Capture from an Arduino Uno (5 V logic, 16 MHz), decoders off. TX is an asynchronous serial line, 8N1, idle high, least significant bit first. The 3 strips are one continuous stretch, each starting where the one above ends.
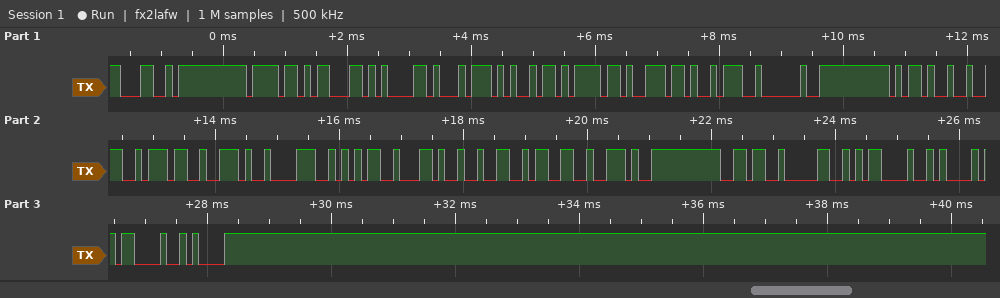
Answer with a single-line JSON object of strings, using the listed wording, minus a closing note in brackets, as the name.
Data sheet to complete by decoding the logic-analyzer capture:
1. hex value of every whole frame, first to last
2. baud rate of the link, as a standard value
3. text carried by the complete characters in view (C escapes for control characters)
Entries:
{"hex value of every whole frame, first to last": "0x4C 0x6F 0x63 0x61 0x74 0x69 0x6F 0x6E 0x3A 0x20 0x2D 0x32 0x37 0x2E 0x38 0x35 0x2C 0x32 0x33 0x2E 0x36 0x30 0x0D 0x0A 0x0D 0x0A", "baud rate of the link, as a standard value": "9600 baud", "text carried by the complete characters in view": "\"Location: -27.85,23.60\\r\\n\\r\\n\""}
